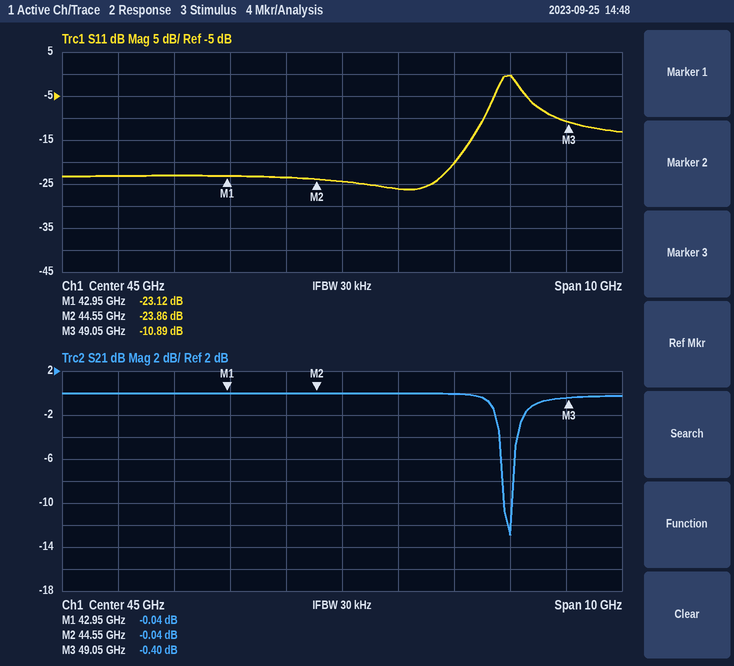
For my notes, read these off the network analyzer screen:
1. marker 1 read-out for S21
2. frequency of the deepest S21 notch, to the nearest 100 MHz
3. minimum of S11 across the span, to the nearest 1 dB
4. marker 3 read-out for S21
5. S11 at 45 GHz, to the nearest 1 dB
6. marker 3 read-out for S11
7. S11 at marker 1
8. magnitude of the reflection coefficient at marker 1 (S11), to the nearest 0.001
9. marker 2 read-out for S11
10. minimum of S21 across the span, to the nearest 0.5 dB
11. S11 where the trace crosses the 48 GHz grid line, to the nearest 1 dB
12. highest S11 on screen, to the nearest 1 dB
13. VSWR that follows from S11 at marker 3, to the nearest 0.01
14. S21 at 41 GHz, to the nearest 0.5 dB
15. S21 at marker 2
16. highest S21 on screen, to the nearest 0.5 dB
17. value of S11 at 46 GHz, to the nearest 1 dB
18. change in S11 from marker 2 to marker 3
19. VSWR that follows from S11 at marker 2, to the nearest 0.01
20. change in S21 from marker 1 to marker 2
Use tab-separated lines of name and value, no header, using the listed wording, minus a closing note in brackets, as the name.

marker 1 read-out for S21	-0.04 dB
frequency of the deepest S21 notch, to the nearest 100 MHz	48.0 GHz
minimum of S11 across the span, to the nearest 1 dB	-26 dB
marker 3 read-out for S21	-0.40 dB
S11 at 45 GHz, to the nearest 1 dB	-24 dB
marker 3 read-out for S11	-10.89 dB
S11 at marker 1	-23.12 dB
magnitude of the reflection coefficient at marker 1 (S11), to the nearest 0.001	0.070
marker 2 read-out for S11	-23.86 dB
minimum of S21 across the span, to the nearest 0.5 dB	-13.0 dB
S11 where the trace crosses the 48 GHz grid line, to the nearest 1 dB	0 dB
highest S11 on screen, to the nearest 1 dB	0 dB
VSWR that follows from S11 at marker 3, to the nearest 0.01	1.80
S21 at 41 GHz, to the nearest 0.5 dB	0.0 dB
S21 at marker 2	-0.04 dB
highest S21 on screen, to the nearest 0.5 dB	0.0 dB
value of S11 at 46 GHz, to the nearest 1 dB	-26 dB
change in S11 from marker 2 to marker 3	12.97 dB
VSWR that follows from S11 at marker 2, to the nearest 0.01	1.14
change in S21 from marker 1 to marker 2	0.00 dB
